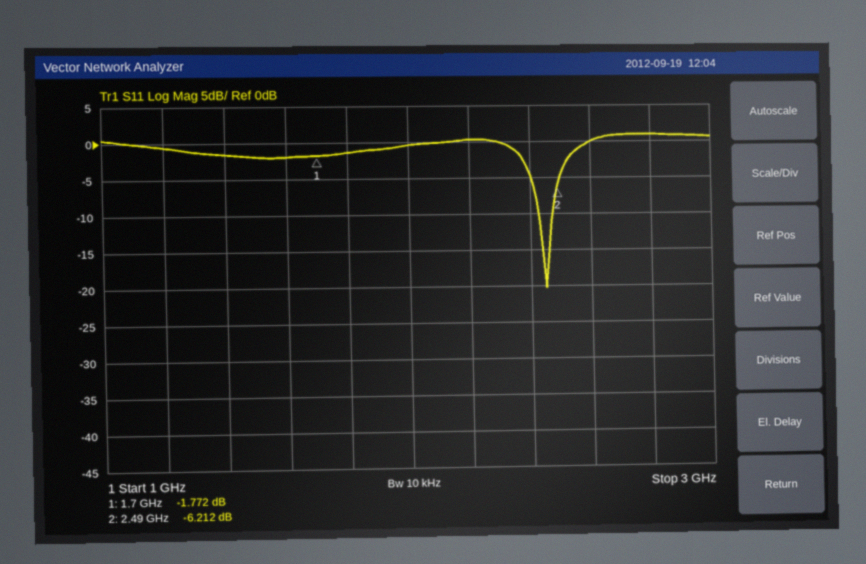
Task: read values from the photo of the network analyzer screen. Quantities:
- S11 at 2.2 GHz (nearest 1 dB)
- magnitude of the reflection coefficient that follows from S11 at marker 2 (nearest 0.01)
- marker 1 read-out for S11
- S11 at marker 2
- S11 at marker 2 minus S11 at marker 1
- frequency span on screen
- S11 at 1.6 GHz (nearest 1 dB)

0 dB
0.49
-1.772 dB
-6.212 dB
-4.440 dB
2 GHz
-2 dB
